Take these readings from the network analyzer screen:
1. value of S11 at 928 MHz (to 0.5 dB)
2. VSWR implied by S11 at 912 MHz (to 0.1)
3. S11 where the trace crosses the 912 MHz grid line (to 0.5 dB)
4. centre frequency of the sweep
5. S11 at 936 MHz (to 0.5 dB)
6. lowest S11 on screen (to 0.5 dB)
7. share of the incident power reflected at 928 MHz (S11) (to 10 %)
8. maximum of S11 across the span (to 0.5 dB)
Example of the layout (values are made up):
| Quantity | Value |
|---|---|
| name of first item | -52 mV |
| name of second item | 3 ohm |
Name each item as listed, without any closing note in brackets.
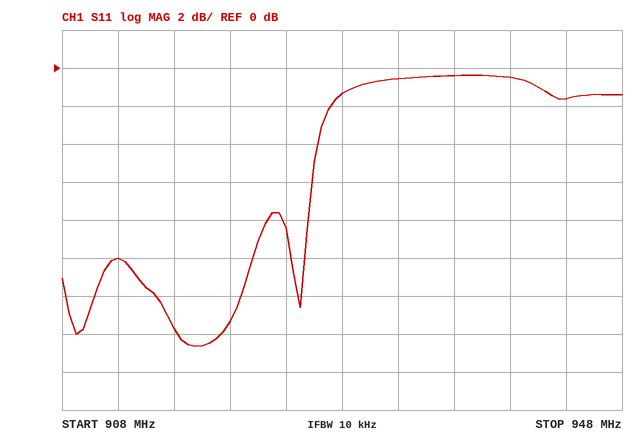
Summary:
| Quantity | Value |
|---|---|
| value of S11 at 928 MHz | -1.5 dB |
| VSWR implied by S11 at 912 MHz | 1.9 |
| S11 where the trace crosses the 912 MHz grid line | -10.0 dB |
| centre frequency of the sweep | 928 MHz |
| S11 at 936 MHz | -0.5 dB |
| lowest S11 on screen | -14.5 dB |
| share of the incident power reflected at 928 MHz (S11) | 70 % |
| maximum of S11 across the span | -0.5 dB |
